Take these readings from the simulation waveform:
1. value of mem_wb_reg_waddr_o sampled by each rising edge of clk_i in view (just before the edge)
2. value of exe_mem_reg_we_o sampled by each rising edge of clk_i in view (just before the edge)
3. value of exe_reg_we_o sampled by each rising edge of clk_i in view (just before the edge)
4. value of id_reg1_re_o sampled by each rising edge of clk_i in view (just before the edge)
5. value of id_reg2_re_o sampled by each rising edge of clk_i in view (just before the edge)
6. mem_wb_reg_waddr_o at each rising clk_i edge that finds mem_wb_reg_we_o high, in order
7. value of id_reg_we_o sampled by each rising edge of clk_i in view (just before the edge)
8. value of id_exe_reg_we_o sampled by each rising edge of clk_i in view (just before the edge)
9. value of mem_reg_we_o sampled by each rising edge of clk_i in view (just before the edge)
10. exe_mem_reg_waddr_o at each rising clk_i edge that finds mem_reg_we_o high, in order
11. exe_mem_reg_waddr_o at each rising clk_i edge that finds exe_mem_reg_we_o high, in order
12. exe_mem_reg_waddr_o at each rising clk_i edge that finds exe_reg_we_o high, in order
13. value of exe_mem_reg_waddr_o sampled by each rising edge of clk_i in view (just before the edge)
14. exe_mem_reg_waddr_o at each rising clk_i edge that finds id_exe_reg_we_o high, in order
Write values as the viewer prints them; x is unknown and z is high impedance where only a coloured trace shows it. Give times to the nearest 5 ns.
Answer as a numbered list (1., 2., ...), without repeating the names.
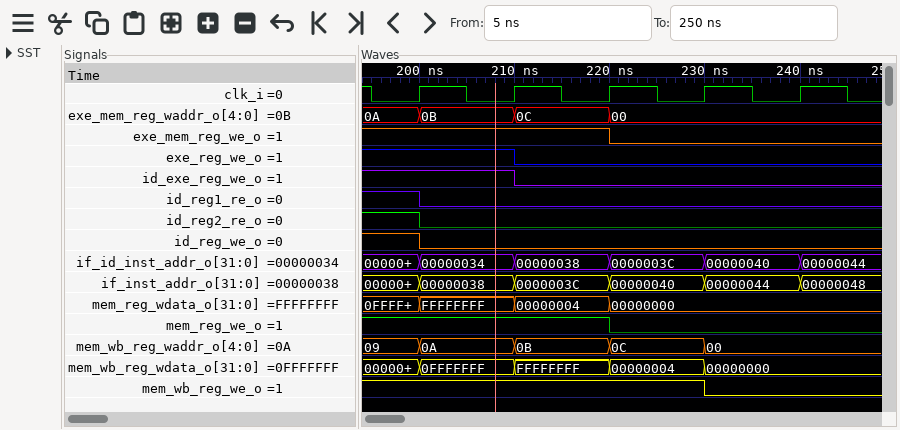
1. 09, 0A, 0B, 0C, 00
2. 1 1 1 0 0
3. 1 1 0 0 0
4. 1 0 0 0 0
5. 1 0 0 0 0
6. 09, 0A, 0B, 0C
7. 1 0 0 0 0
8. 1 1 0 0 0
9. 1 1 1 0 0
10. 0A, 0B, 0C
11. 0A, 0B, 0C
12. 0A, 0B
13. 0A, 0B, 0C, 00, 00
14. 0A, 0B
